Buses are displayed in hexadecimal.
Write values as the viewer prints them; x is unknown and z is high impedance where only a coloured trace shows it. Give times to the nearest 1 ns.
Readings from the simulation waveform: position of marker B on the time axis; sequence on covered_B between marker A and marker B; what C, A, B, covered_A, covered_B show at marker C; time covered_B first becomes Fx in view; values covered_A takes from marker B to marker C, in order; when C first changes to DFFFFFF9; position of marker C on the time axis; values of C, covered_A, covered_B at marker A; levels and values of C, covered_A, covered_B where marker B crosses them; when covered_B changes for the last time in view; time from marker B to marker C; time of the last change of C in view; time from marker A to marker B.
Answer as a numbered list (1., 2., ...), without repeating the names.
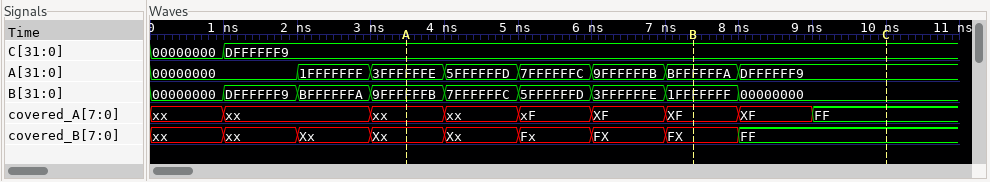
1. 7 ns
2. Xx, Xx, Fx, FX, FX
3. C=DFFFFFF9, A=DFFFFFF9, B=00000000, covered_A=FF, covered_B=FF
4. 5 ns
5. XF, XF, FF
6. 1 ns
7. 10 ns
8. C=DFFFFFF9, covered_A=xx, covered_B=Xx
9. C=DFFFFFF9, covered_A=XF, covered_B=FX
10. 8 ns
11. 3 ns
12. 1 ns
13. 4 ns
